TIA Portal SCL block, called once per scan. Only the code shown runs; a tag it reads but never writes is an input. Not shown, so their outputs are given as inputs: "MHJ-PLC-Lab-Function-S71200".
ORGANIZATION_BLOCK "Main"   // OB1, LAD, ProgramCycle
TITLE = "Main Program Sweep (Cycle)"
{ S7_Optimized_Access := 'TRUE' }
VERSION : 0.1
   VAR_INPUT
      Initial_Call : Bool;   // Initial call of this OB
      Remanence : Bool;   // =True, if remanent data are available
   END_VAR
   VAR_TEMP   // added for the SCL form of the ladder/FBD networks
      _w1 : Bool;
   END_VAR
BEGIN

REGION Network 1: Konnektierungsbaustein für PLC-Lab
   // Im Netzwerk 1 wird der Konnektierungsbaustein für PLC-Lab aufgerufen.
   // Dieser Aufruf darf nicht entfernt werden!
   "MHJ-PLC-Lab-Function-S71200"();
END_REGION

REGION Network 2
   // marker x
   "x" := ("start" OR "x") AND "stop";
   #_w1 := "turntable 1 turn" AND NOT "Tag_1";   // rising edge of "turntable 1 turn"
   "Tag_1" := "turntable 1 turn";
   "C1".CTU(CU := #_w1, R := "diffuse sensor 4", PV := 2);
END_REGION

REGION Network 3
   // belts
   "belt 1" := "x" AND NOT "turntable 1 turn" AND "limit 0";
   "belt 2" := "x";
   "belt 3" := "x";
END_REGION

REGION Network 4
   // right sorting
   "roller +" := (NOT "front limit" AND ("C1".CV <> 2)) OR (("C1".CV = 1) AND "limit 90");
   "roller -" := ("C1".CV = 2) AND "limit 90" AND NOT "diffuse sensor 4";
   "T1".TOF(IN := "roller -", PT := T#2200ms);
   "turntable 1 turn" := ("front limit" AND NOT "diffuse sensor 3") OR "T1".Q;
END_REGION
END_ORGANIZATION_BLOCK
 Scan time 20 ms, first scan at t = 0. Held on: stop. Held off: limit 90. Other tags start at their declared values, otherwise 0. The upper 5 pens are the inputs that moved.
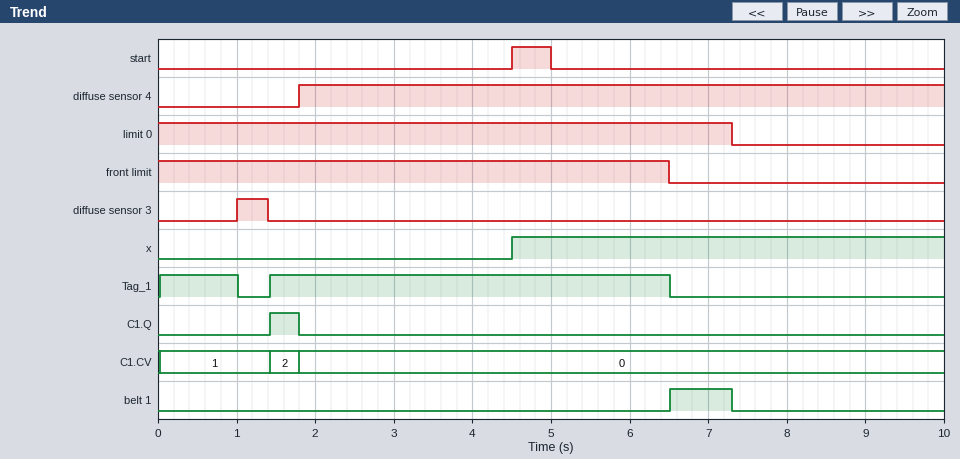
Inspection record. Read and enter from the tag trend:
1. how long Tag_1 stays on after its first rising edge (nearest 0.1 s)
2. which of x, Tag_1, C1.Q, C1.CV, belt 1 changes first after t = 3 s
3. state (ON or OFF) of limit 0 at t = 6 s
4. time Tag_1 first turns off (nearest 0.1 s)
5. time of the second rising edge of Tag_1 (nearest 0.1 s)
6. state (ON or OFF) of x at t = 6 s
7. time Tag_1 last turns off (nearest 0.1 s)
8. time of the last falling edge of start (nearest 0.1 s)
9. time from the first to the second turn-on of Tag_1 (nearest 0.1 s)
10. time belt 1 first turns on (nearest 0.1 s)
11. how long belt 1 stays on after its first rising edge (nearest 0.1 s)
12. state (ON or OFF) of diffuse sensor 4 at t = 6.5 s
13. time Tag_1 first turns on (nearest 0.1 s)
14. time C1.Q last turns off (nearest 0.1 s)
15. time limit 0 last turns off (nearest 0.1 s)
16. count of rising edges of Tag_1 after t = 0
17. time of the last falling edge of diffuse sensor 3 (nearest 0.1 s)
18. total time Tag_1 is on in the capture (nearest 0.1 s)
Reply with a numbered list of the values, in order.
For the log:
1. 1.0 s
2. x
3. ON
4. 1.0 s
5. 1.4 s
6. ON
7. 6.5 s
8. 5.0 s
9. 1.4 s
10. 6.5 s
11. 0.8 s
12. ON
13. 0.0 s
14. 1.8 s
15. 7.3 s
16. 2
17. 1.4 s
18. 6.1 s
